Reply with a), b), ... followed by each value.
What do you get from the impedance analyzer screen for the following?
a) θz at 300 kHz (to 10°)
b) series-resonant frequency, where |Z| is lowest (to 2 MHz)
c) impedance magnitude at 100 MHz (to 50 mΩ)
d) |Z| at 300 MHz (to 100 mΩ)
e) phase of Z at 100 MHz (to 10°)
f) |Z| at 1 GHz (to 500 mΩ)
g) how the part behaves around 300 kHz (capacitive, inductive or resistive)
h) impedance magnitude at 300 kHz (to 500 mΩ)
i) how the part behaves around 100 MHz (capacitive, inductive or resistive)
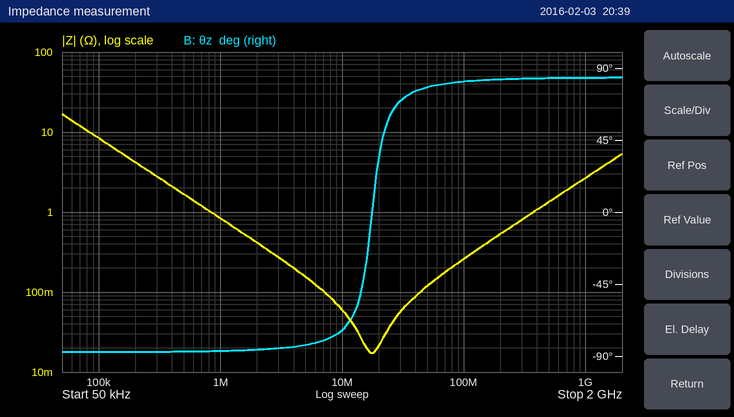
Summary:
a) -90°
b) 18 MHz
c) 250 mΩ
d) 800 mΩ
e) 80°
f) 2.5 Ω
g) capacitive
h) 3.0 Ω
i) inductive
